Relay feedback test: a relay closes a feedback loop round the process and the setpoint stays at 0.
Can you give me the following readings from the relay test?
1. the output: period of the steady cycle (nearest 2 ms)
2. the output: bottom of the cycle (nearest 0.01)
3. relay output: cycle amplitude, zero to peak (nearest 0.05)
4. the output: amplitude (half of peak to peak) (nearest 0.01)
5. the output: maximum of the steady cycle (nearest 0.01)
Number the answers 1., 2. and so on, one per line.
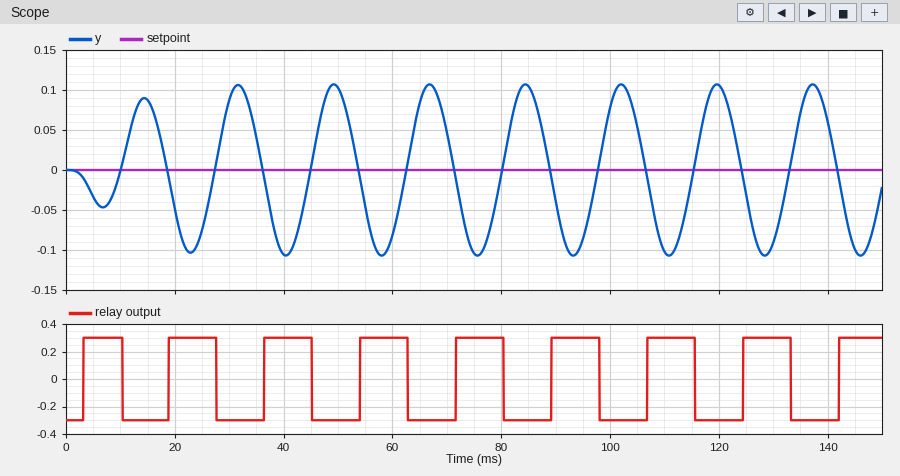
1. 18 ms
2. -0.11
3. 0.30
4. 0.11
5. 0.11
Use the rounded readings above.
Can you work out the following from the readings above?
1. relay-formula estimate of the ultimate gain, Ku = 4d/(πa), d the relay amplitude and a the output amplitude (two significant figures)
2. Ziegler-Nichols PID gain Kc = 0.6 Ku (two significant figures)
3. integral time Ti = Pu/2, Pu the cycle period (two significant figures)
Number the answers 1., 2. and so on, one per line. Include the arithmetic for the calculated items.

1. 4 × 0.3 / (π × 0.11) = 3.5
2. 0.6 × 3.5 = 2.1
3. 18 / 2 = 9.0 ms
